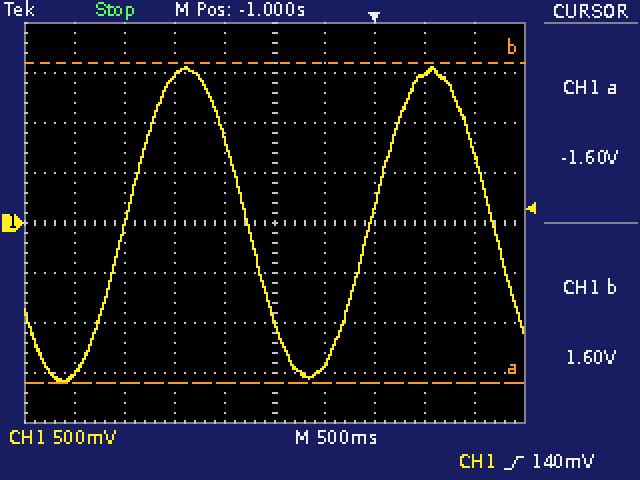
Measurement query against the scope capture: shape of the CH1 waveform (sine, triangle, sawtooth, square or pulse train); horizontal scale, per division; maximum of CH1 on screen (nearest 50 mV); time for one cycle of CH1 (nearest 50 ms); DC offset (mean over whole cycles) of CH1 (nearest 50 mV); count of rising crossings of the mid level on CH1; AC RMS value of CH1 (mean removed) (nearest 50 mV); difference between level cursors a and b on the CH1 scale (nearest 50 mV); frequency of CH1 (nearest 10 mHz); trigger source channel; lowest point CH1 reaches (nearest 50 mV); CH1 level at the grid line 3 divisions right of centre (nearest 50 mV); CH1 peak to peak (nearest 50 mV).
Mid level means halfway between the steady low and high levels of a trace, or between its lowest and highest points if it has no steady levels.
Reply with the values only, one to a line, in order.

sine
500 ms
1.55 V
2.45 s
0 mV
2
1.10 V
3.20 V
410 mHz
CH1
-1.60 V
1.50 V
3.15 V
